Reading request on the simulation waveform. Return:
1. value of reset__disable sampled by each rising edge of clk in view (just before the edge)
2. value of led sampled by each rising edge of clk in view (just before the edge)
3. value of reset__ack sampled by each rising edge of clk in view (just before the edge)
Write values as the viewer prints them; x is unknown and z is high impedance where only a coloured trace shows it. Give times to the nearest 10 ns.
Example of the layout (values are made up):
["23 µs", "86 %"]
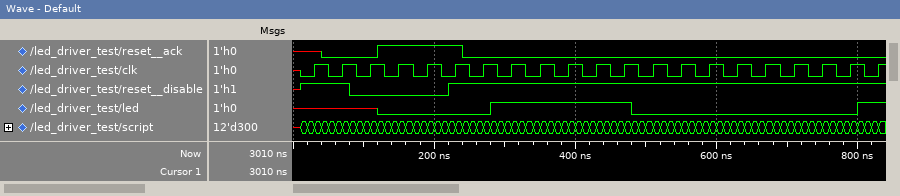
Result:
["1 1 0 0 0 1 1 1 1 1 1 1 1 1 1 1 1 1 1 1 1", "x x x 0 0 0 0 1 1 1 1 1 0 0 0 0 0 0 0 0 1", "x 0 0 1 1 1 0 0 0 0 0 0 0 0 0 0 0 0 0 0 0"]
